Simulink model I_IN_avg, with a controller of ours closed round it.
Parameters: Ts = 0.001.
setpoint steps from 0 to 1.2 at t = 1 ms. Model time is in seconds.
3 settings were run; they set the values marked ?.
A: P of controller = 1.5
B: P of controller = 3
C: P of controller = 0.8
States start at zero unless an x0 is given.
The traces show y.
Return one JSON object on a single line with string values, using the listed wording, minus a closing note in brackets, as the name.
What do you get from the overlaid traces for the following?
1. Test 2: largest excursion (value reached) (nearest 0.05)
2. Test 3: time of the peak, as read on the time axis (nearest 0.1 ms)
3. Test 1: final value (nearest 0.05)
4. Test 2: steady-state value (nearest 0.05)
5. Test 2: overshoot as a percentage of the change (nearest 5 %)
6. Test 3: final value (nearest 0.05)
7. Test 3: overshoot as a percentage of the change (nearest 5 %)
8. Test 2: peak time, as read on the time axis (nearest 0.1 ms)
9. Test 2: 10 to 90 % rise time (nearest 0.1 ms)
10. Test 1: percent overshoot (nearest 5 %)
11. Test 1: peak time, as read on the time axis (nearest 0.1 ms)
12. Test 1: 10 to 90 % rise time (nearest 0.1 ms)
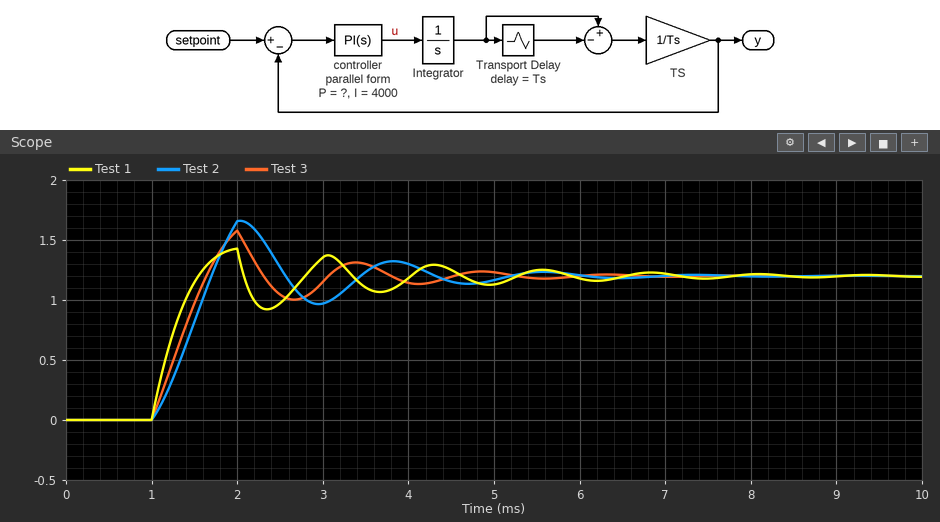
{"Test 2: largest excursion (value reached)": "1.65", "Test 3: time of the peak, as read on the time axis": "2.0 ms", "Test 1: final value": "1.20", "Test 2: steady-state value": "1.20", "Test 2: overshoot as a percentage of the change": "40 %", "Test 3: final value": "1.20", "Test 3: overshoot as a percentage of the change": "30 %", "Test 2: peak time, as read on the time axis": "2.0 ms", "Test 2: 10 to 90 % rise time": "0.5 ms", "Test 1: percent overshoot": "20 %", "Test 1: peak time, as read on the time axis": "2.0 ms", "Test 1: 10 to 90 % rise time": "0.4 ms"}
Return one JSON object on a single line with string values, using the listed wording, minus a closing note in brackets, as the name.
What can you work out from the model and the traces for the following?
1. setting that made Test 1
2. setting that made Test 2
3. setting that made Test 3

{"setting that made Test 1": "B", "setting that made Test 2": "C", "setting that made Test 3": "A"}
